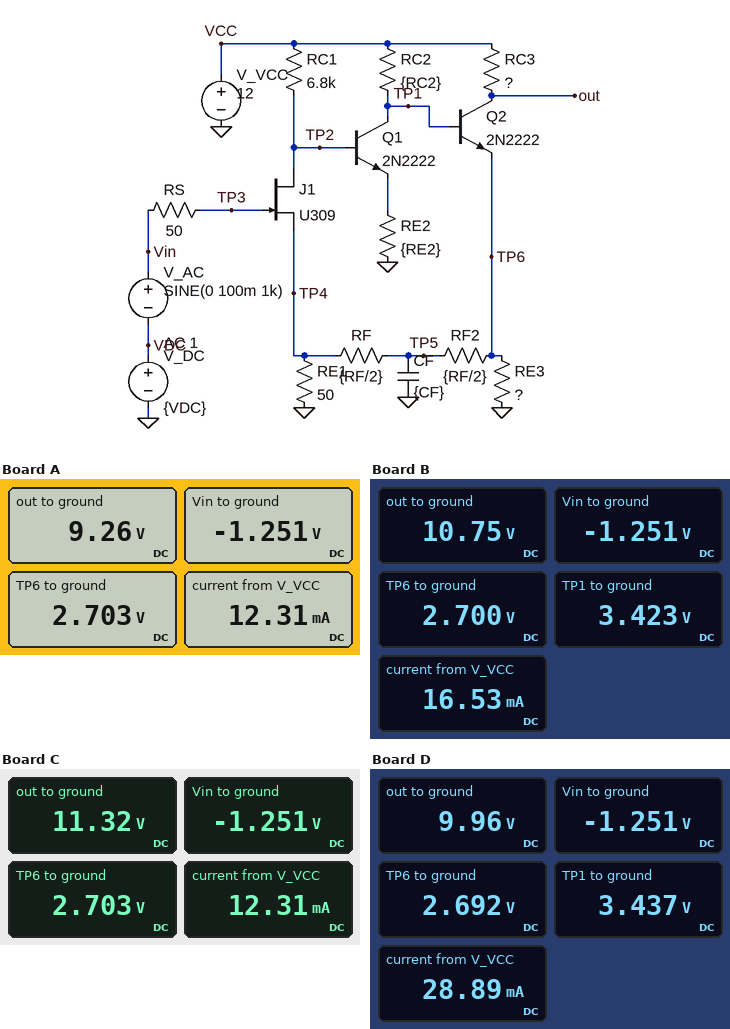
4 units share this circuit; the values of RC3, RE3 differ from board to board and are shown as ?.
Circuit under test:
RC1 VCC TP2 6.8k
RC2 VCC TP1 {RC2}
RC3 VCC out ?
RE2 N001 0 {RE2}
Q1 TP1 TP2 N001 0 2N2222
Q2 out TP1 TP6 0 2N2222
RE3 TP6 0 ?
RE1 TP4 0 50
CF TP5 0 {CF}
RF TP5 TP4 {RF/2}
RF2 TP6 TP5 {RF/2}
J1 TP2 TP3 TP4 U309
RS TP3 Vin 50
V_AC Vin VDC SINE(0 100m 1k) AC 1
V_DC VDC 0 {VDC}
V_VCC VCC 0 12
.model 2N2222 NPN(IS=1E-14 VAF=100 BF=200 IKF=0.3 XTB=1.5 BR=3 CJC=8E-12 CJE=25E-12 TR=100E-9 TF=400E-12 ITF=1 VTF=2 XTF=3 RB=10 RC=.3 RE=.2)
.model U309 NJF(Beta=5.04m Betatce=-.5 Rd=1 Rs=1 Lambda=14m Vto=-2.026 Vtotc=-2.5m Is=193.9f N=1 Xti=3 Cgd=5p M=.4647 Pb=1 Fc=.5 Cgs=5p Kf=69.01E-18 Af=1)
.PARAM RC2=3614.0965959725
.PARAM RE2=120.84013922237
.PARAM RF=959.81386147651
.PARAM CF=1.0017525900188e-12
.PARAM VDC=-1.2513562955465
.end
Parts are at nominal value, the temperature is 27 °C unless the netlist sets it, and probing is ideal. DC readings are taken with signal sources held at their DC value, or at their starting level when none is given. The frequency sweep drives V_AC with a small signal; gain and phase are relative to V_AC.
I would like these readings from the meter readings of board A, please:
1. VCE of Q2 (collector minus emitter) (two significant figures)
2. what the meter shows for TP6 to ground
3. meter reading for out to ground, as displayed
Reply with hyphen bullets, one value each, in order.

- 6.6 V
- 2.703 V
- 9.26 V
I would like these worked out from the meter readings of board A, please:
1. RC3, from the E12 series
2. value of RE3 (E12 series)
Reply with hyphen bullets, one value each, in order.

- 330 Ω
- 470 Ω
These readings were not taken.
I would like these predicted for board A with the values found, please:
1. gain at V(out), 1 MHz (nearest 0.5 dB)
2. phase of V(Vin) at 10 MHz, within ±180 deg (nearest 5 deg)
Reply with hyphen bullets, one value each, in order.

- 26.0 dB
- 0 deg
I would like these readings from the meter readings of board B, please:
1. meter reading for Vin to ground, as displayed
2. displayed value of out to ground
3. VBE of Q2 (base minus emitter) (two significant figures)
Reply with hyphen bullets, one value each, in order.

- -1.251 V
- 10.75 V
- 720 mV
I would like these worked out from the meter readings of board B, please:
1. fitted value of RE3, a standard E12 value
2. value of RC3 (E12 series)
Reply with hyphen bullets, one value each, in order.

- 270 Ω
- 100 Ω
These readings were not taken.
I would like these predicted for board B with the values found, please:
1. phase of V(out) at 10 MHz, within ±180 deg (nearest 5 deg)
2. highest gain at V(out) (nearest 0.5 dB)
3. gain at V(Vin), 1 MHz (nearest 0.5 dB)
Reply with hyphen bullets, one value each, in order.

- 100 deg
- 19.0 dB
- 0 dB
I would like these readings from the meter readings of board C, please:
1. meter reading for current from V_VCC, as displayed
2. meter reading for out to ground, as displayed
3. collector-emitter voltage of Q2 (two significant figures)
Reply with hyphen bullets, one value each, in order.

- 12.31 mA
- 11.32 V
- 8.6 V
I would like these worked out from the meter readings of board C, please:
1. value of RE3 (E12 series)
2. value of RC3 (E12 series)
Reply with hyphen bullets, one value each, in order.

- 470 Ω
- 82 Ω
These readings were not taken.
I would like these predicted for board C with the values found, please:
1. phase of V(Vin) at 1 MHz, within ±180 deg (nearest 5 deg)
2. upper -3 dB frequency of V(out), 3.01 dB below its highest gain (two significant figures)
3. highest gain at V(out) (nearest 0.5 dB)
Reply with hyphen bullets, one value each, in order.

- 0 deg
- 7.6 MHz
- 14.0 dB
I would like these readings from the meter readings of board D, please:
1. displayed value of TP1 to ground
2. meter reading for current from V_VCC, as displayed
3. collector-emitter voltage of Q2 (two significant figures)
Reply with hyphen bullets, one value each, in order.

- 3.437 V
- 28.89 mA
- 7.3 V
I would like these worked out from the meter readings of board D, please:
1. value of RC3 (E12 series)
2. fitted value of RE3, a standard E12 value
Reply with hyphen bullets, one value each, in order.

- 82 Ω
- 120 Ω
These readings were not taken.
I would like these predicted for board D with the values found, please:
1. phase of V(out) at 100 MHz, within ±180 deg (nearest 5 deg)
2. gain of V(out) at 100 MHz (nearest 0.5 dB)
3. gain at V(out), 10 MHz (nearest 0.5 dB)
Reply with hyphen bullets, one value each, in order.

- -75 deg
- -7.5 dB
- 19.0 dB
